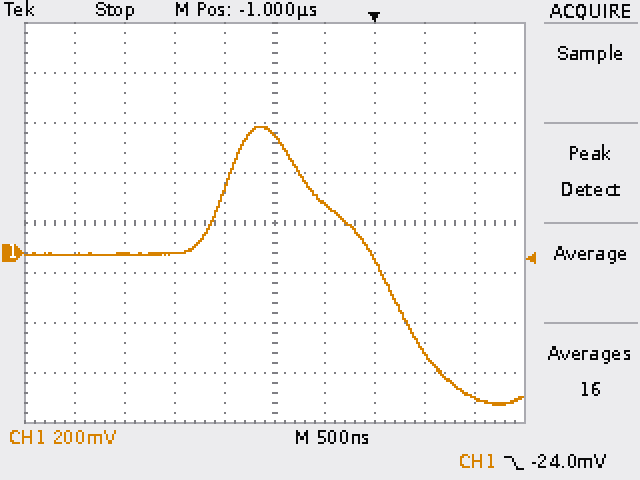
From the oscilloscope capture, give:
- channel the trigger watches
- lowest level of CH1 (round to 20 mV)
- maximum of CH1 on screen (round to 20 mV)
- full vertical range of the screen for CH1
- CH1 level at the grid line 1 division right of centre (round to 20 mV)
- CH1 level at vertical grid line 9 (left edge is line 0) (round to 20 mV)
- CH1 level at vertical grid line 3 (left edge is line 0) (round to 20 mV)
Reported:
CH1
-600 mV
500 mV
1.6 V
200 mV
-580 mV
0 mV
